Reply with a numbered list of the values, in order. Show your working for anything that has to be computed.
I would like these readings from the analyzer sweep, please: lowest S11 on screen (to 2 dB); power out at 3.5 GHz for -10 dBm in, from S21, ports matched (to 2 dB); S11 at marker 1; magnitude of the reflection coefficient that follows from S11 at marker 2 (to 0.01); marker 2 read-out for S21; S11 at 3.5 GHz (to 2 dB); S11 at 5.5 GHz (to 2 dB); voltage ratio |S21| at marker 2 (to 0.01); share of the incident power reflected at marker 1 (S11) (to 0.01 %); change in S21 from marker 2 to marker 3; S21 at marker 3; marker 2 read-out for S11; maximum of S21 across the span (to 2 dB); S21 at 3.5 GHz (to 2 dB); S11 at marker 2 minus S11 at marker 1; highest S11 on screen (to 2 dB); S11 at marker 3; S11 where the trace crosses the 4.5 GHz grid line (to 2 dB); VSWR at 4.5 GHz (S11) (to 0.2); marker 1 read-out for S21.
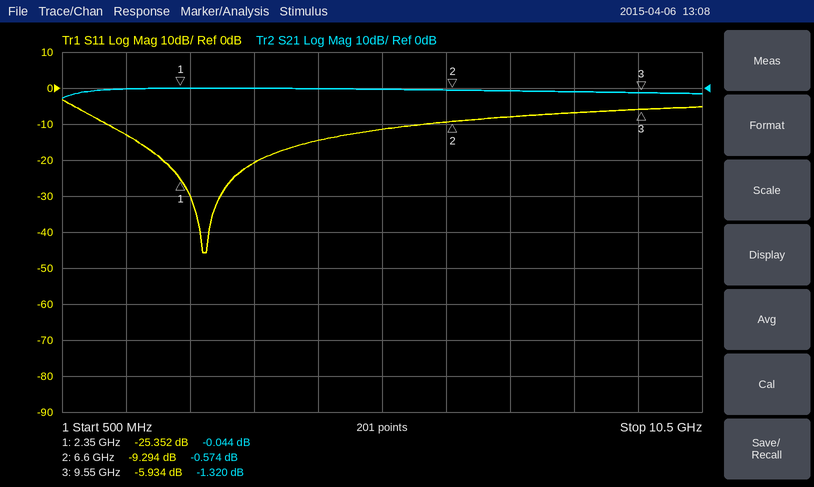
1. -46 dB
2. -10 dBm + (0 dB) = -10 dBm
3. -25.352 dB
4. 10^(-9.294/20) ≈ 0.34
5. -0.574 dB
6. -20 dB
7. -12 dB
8. 10^(-0.574/20) ≈ 0.94
9. 10^(-25.352/10) ≈ 0.29 %
10. -1.32 − (-0.574) = -0.746 dB
11. -1.320 dB
12. -9.294 dB
13. 0 dB
14. 0 dB
15. -9.294 − (-25.352) = 16.058 dB
16. -4 dB
17. -5.934 dB
18. -14 dB
19. |Γ| = 10^(-14/20) = 0.1995; VSWR = (1 + 0.1995)/(1 − 0.1995) ≈ 1.50, so 1.4 to the nearest 0.2
20. -0.044 dB
